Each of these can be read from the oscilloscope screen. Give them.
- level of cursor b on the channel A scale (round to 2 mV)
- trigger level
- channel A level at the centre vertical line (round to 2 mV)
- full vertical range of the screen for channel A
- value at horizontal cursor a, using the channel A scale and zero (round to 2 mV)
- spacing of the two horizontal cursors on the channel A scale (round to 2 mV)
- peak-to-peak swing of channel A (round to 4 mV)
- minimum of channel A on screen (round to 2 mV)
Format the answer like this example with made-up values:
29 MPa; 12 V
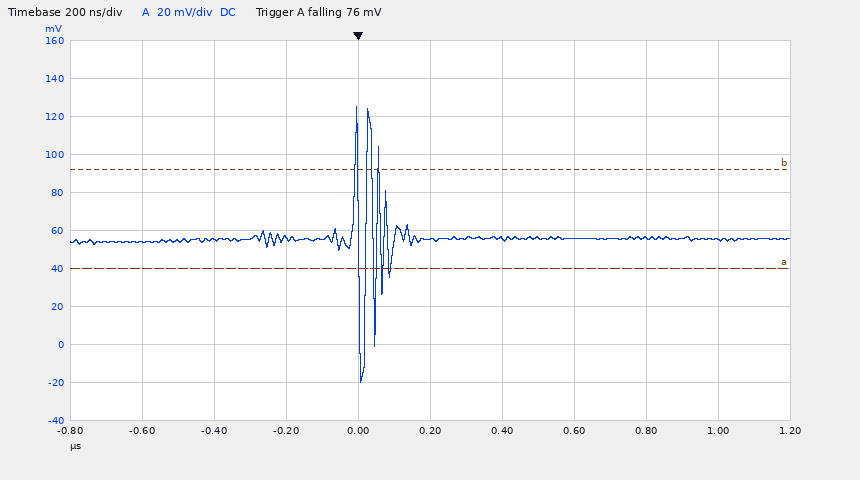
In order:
92 mV; 76 mV; 56 mV; 200 mV; 40 mV; 52 mV; 144 mV; -20 mV
